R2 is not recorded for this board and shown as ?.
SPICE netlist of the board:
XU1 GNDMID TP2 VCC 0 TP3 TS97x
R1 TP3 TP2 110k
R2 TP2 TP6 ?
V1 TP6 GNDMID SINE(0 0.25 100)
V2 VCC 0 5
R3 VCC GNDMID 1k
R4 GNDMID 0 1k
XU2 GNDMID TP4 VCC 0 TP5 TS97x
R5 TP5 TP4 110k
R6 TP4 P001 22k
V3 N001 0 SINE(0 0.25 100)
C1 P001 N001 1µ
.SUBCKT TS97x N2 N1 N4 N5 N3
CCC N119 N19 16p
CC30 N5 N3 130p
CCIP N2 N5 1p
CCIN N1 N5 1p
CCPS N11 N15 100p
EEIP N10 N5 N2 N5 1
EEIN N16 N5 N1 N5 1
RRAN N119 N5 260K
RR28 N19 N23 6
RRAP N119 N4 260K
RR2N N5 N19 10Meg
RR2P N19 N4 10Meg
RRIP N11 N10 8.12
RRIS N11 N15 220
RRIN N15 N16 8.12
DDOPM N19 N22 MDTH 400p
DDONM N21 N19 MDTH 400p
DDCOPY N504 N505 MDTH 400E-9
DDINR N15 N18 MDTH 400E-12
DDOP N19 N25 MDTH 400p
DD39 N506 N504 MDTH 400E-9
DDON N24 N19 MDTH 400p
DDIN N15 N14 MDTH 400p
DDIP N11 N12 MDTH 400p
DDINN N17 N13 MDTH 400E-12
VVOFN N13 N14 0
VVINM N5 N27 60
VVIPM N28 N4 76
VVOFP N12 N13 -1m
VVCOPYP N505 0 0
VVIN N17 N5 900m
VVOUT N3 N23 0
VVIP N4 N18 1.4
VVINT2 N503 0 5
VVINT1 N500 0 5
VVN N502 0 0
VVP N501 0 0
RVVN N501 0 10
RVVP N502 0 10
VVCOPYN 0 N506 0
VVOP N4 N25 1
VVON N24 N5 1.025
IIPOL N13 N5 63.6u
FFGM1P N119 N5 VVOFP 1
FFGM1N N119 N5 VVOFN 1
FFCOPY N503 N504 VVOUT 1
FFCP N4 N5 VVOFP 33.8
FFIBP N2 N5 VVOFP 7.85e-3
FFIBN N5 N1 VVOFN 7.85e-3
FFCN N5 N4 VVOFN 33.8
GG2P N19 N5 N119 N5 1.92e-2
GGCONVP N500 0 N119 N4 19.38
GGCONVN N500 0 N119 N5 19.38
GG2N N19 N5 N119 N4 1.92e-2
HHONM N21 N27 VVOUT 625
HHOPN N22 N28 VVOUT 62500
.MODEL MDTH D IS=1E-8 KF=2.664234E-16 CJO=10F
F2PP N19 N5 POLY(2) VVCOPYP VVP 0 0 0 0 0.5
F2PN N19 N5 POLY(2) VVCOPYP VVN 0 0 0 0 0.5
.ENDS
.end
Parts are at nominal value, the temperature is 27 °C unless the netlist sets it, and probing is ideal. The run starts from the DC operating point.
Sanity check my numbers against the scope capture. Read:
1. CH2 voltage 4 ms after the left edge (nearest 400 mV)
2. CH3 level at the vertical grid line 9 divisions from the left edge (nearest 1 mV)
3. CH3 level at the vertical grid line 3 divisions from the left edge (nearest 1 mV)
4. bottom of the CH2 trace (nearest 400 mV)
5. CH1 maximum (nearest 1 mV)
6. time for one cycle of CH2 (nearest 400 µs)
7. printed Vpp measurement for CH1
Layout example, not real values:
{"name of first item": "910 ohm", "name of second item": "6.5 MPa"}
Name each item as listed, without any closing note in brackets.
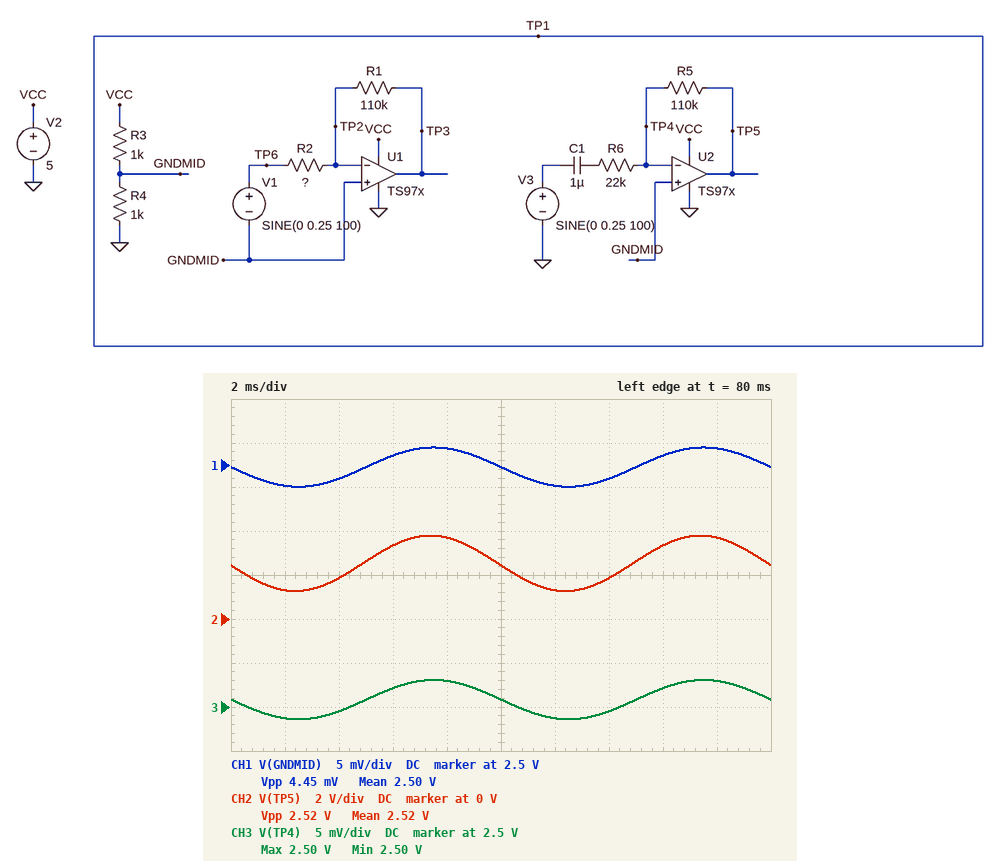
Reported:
{"CH2 voltage 4 ms after the left edge": "2.0 V", "CH3 level at the vertical grid line 9 divisions from the left edge": "2.503 V", "CH3 level at the vertical grid line 3 divisions from the left edge": "2.502 V", "bottom of the CH2 trace": "1.2 V", "CH1 maximum": "2.502 V", "time for one cycle of CH2": "10.0 ms", "printed Vpp measurement for CH1": "4.45 mV"}
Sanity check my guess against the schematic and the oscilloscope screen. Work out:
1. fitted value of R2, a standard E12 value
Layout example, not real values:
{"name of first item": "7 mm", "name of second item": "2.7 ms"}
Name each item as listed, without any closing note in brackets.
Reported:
{"fitted value of R2, a standard E12 value": "56 kΩ"}
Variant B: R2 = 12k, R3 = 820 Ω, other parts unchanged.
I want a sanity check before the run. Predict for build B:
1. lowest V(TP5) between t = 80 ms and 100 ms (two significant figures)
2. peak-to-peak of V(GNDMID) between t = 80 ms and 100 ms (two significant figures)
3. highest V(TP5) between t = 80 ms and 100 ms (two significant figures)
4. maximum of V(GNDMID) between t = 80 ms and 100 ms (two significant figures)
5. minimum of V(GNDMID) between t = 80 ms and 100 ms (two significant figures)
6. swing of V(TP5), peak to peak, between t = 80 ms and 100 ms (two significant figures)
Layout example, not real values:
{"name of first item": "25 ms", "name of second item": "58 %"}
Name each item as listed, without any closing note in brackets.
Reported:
{"lowest V(TP5) between t = 80 ms and 100 ms": "1.5 V", "peak-to-peak of V(GNDMID) between t = 80 ms and 100 ms": "18 mV", "highest V(TP5) between t = 80 ms and 100 ms": "4.1 V", "maximum of V(GNDMID) between t = 80 ms and 100 ms": "2.8 V", "minimum of V(GNDMID) between t = 80 ms and 100 ms": "2.7 V", "swing of V(TP5), peak to peak, between t = 80 ms and 100 ms": "2.6 V"}
